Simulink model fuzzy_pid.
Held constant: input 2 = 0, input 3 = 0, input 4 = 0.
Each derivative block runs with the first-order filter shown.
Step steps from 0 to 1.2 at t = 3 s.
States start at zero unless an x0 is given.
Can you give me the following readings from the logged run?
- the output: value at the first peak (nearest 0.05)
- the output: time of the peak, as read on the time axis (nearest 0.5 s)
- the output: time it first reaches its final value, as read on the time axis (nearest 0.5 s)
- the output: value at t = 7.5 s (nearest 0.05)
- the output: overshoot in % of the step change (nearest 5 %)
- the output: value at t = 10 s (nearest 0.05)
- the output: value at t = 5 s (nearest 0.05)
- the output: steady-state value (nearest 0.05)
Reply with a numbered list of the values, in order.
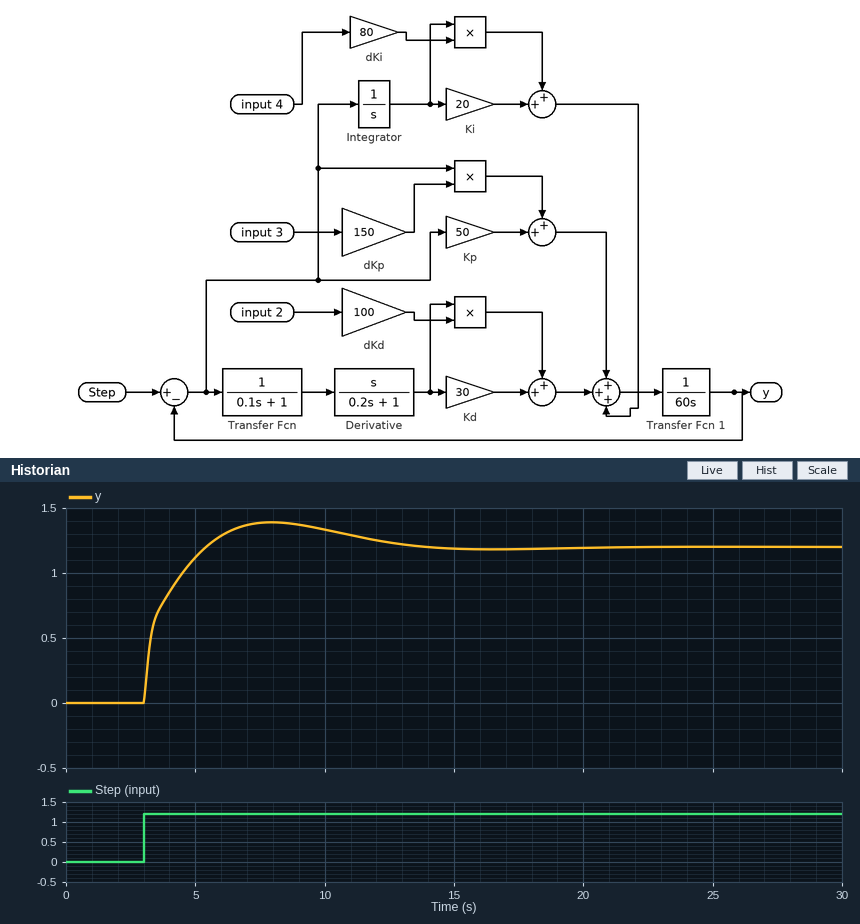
1. 1.40
2. 8.0 s
3. 5.5 s
4. 1.40
5. 15 %
6. 1.35
7. 1.10
8. 1.20
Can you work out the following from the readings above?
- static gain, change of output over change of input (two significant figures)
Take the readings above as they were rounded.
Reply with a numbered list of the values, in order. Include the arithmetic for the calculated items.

1. (1.2 - 0) / (1.2 - 0) = 1.0
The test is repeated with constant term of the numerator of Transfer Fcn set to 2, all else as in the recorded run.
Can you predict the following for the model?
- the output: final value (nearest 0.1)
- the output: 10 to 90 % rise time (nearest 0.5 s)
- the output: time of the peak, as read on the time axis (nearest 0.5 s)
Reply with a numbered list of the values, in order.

1. 1.2
2. 2.0 s
3. 9.0 s
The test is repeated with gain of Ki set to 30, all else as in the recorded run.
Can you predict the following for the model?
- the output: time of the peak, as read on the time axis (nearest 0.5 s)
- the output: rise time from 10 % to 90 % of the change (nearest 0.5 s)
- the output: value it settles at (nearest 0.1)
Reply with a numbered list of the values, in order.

1. 7.0 s
2. 1.5 s
3. 1.2
